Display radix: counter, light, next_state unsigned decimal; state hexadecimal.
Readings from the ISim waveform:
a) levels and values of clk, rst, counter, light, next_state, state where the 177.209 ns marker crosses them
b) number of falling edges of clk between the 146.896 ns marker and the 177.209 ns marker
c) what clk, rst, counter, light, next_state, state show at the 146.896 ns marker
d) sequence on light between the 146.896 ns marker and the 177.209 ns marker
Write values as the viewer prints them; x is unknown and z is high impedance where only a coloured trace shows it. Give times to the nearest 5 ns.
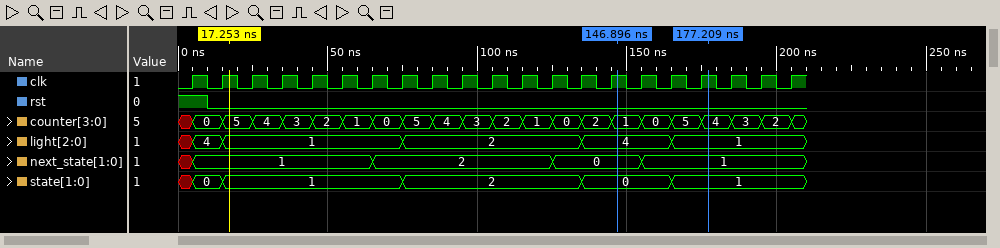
clk=1, rst=0, counter=4, light=1, next_state=1, state=1
3
clk=1, rst=0, counter=1, light=4, next_state=0, state=0
4, 1
